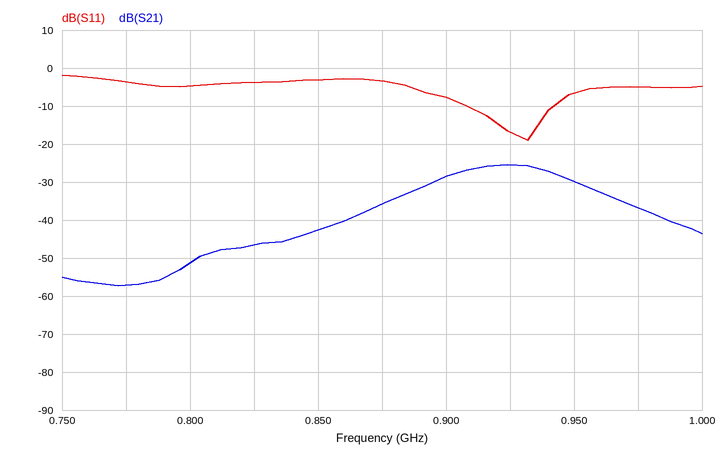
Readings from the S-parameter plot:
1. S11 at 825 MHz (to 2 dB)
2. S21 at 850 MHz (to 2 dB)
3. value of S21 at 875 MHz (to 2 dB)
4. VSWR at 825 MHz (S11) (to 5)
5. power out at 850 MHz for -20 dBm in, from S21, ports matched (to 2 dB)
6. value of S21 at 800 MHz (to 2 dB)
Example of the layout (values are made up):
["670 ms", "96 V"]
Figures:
["-4 dB", "-42 dB", "-36 dB", "5", "-62 dBm", "-52 dB"]
